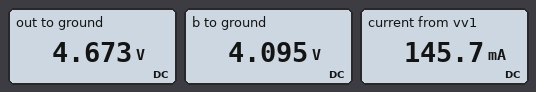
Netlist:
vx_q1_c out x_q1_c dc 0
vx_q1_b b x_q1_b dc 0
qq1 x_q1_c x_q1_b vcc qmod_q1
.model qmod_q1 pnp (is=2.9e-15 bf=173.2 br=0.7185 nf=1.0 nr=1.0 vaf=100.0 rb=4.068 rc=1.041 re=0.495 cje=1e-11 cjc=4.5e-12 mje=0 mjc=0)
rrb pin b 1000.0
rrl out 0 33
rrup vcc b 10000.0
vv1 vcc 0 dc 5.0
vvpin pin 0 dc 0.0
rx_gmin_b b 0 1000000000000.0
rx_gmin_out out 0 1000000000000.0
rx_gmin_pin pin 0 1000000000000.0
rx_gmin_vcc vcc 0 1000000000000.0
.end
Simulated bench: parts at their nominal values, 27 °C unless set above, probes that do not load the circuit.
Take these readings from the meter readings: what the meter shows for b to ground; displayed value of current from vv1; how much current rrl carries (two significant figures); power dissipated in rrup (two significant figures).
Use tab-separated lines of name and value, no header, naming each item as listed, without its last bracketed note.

what the meter shows for b to ground	4.095 V
displayed value of current from vv1	145.7 mA
how much current rrl carries	140 mA
power dissipated in rrup	82 µW
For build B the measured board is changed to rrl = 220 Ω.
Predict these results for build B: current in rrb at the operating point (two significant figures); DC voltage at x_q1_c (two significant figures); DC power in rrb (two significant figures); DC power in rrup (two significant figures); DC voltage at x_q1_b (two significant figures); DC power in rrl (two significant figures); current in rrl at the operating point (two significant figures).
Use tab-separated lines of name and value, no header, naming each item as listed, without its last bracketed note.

current in rrb at the operating point	4.2 mA
DC voltage at x_q1_c	4.9 V
DC power in rrb	18 mW
DC power in rrup	65 µW
DC voltage at x_q1_b	4.2 V
DC power in rrl	110 mW
current in rrl at the operating point	22 mA
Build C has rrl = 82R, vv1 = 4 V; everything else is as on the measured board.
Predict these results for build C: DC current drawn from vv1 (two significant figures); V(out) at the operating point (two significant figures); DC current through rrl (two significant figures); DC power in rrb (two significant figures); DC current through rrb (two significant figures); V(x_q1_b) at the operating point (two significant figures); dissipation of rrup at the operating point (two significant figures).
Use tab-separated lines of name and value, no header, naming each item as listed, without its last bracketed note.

DC current drawn from vv1	50 mA
V(out) at the operating point	3.8 V
DC current through rrl	47 mA
DC power in rrb	10 mW
DC current through rrb	3.2 mA
V(x_q1_b) at the operating point	3.2 V
dissipation of rrup at the operating point	68 µW
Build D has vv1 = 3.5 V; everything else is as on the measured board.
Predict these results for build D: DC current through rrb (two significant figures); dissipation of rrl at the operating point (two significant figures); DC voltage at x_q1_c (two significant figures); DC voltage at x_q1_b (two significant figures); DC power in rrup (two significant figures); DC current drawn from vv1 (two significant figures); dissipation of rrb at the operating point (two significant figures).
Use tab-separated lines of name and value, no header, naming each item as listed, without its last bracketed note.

DC current through rrb	2.6 mA
dissipation of rrl at the operating point	320 mW
DC voltage at x_q1_c	3.2 V
DC voltage at x_q1_b	2.6 V
DC power in rrup	75 µW
DC current drawn from vv1	100 mA
dissipation of rrb at the operating point	6.9 mW
